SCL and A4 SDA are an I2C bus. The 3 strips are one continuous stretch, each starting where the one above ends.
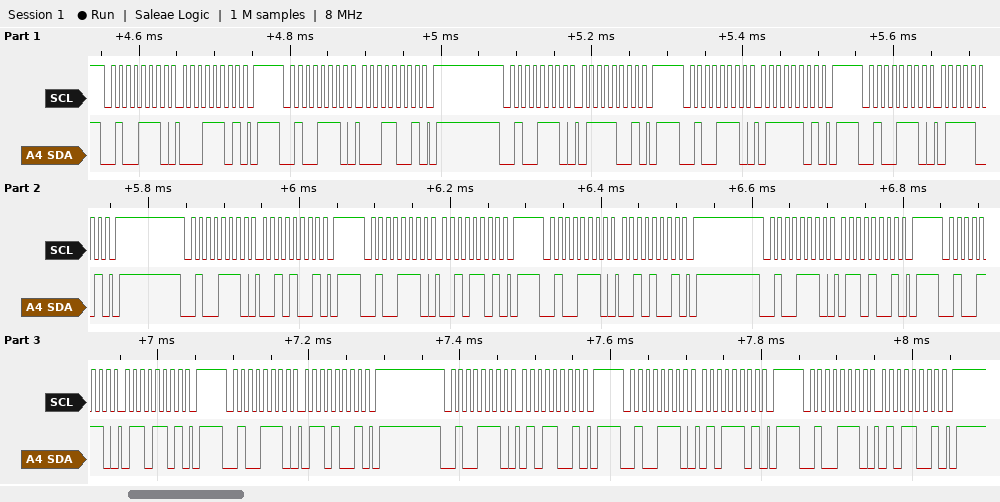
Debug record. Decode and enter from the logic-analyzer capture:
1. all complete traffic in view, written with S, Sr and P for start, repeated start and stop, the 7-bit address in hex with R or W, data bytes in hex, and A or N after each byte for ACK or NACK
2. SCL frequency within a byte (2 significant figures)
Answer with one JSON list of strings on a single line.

["S 27W A 1D A P S 27W A 19 A P S 27W A 79 A P S 27W A 7D A P S 27W A 79 A P S 27W A 29 A P S 27W A 2D A P S 27W A 29 A P S 27W A 69 A P S 27W A 6D A P S 27W A 69 A P S 27W A 59 A P S 27W A 5D A P S 27W A 59 A P", "100 kHz"]
